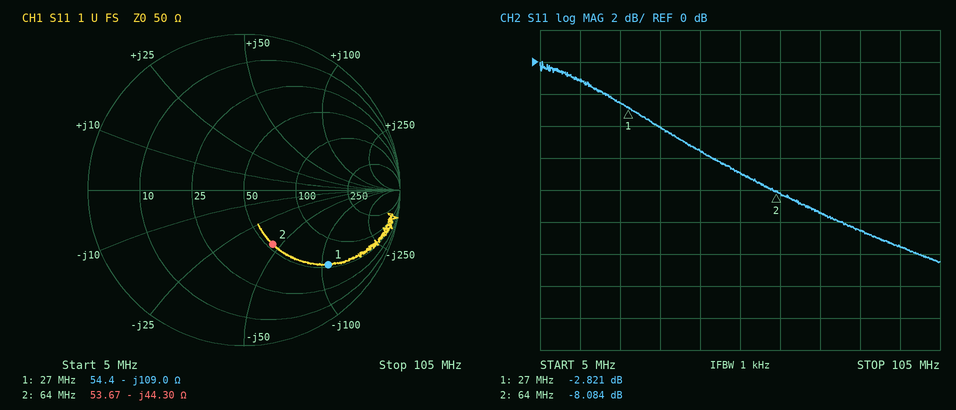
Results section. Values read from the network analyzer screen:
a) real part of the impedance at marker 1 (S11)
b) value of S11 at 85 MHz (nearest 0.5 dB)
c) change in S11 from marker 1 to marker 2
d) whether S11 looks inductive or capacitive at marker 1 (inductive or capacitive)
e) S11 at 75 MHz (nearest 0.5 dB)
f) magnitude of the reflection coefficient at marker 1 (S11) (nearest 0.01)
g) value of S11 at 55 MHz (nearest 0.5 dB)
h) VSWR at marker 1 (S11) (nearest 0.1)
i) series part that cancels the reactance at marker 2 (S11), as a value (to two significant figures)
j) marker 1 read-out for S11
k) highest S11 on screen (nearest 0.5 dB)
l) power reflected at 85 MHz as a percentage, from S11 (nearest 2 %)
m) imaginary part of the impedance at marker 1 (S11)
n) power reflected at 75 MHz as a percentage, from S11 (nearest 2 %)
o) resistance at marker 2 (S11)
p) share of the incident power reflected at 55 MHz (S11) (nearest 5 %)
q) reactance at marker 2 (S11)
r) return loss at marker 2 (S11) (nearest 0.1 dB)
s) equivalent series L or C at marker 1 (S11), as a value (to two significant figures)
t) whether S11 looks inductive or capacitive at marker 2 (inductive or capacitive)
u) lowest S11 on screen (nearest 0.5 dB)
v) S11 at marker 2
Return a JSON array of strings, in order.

["54.4 Ω", "-10.5 dB", "-5.263 dB", "capacitive", "-9.5 dB", "0.72", "-7.0 dB", "6.2", "110 nH", "-2.821 dB", "0.0 dB", "8 %", "-109.0 Ω", "12 %", "53.67 Ω", "20 %", "-44.30 Ω", "8.1 dB", "54 pF", "capacitive", "-12.5 dB", "-8.084 dB"]
